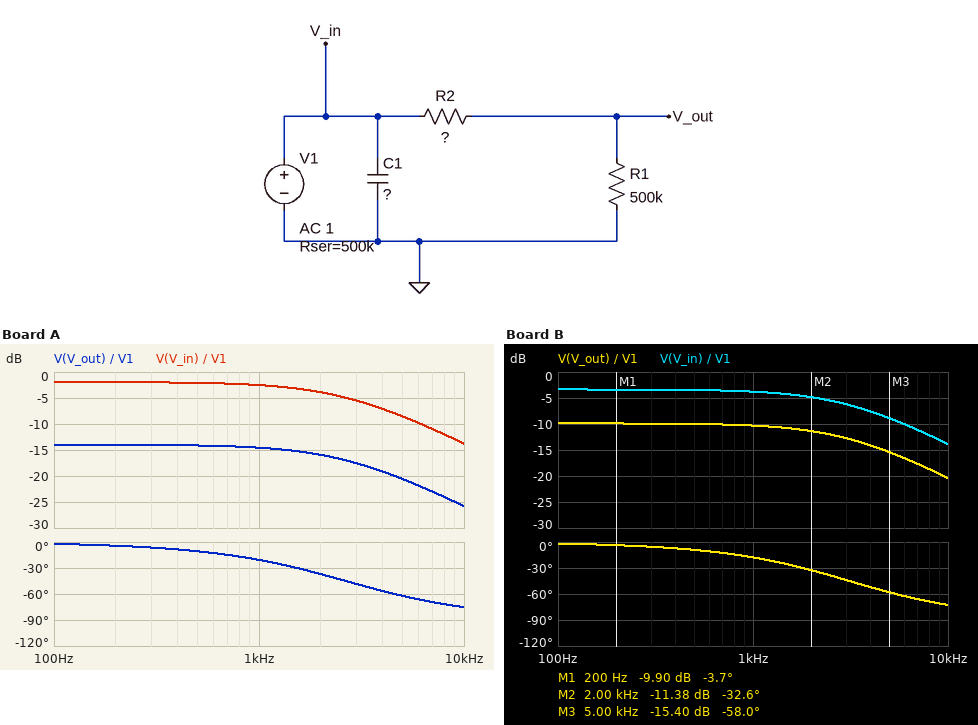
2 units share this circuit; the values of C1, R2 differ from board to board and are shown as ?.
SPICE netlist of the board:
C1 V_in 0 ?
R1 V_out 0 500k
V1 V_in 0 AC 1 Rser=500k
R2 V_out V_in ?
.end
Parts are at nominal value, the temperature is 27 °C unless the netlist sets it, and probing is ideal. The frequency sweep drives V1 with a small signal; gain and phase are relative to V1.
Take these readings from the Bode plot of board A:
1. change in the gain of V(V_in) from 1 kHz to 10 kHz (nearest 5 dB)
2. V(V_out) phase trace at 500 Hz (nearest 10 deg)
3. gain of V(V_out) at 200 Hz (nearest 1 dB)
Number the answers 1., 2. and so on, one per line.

1. -10 dB
2. -10 deg
3. -14 dB
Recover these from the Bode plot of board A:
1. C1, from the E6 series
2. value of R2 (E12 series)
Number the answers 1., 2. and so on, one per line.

1. 150 pF
2. 1.5 MΩ
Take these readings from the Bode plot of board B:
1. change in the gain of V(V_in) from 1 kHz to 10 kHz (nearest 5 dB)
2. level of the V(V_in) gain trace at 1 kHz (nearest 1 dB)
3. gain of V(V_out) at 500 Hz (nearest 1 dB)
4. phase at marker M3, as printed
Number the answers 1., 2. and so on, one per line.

1. -10 dB
2. -4 dB
3. -10 dB
4. -58.0 deg
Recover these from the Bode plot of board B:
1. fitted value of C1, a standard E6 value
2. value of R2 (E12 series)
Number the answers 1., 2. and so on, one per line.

1. 150 pF
2. 560 kΩ
